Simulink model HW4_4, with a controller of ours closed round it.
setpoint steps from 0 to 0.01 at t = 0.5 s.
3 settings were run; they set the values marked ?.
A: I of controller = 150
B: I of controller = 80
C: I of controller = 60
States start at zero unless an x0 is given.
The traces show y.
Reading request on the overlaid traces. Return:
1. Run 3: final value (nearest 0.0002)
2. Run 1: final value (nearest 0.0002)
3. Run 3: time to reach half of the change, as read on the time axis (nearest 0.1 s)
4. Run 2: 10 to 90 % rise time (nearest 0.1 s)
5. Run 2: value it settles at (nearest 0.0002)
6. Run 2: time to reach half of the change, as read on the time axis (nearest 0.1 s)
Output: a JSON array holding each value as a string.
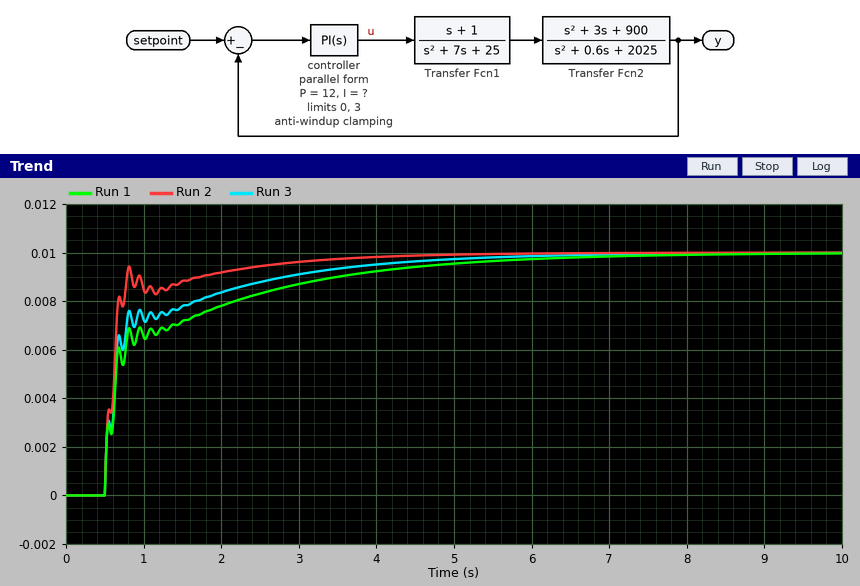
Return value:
["0.0100", "0.0100", "0.6 s", "0.3 s", "0.0100", "0.6 s"]
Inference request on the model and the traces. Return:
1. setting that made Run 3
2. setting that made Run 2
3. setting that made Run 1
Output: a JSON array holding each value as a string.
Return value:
["B", "A", "C"]
